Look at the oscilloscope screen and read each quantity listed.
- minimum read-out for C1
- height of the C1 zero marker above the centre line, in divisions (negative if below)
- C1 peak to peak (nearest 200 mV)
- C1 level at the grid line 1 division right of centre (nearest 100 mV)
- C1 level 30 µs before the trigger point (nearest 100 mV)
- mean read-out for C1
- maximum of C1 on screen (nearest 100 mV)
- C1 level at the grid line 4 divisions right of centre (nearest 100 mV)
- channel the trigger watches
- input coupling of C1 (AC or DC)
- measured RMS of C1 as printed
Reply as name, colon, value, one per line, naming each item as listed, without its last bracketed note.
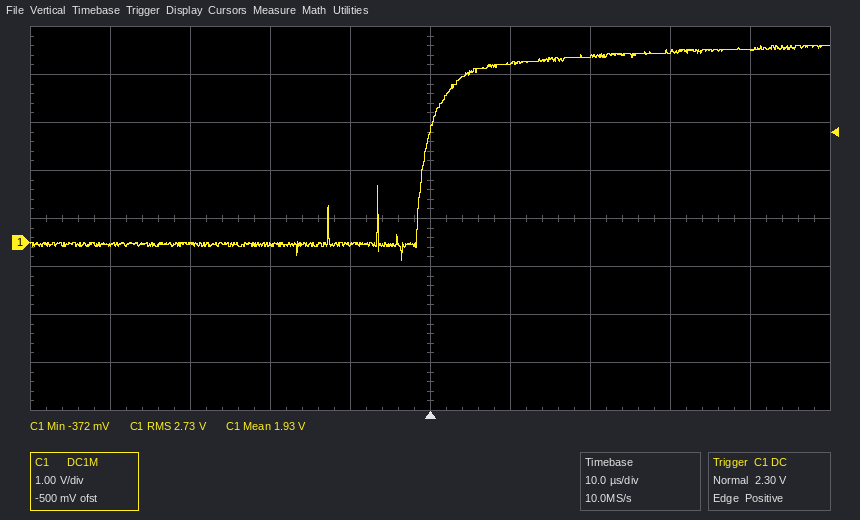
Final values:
minimum read-out for C1: -372 mV
height of the C1 zero marker above the centre line, in divisions: -0.5 div
C1 peak to peak: 4.4 V
C1 level at the grid line 1 division right of centre: 3.7 V
C1 level 30 µs before the trigger point: 0.0 V
mean read-out for C1: 1.93 V
maximum of C1 on screen: 4.1 V
C1 level at the grid line 4 divisions right of centre: 4.0 V
channel the trigger watches: C1
input coupling of C1: DC
measured RMS of C1 as printed: 2.73 V
